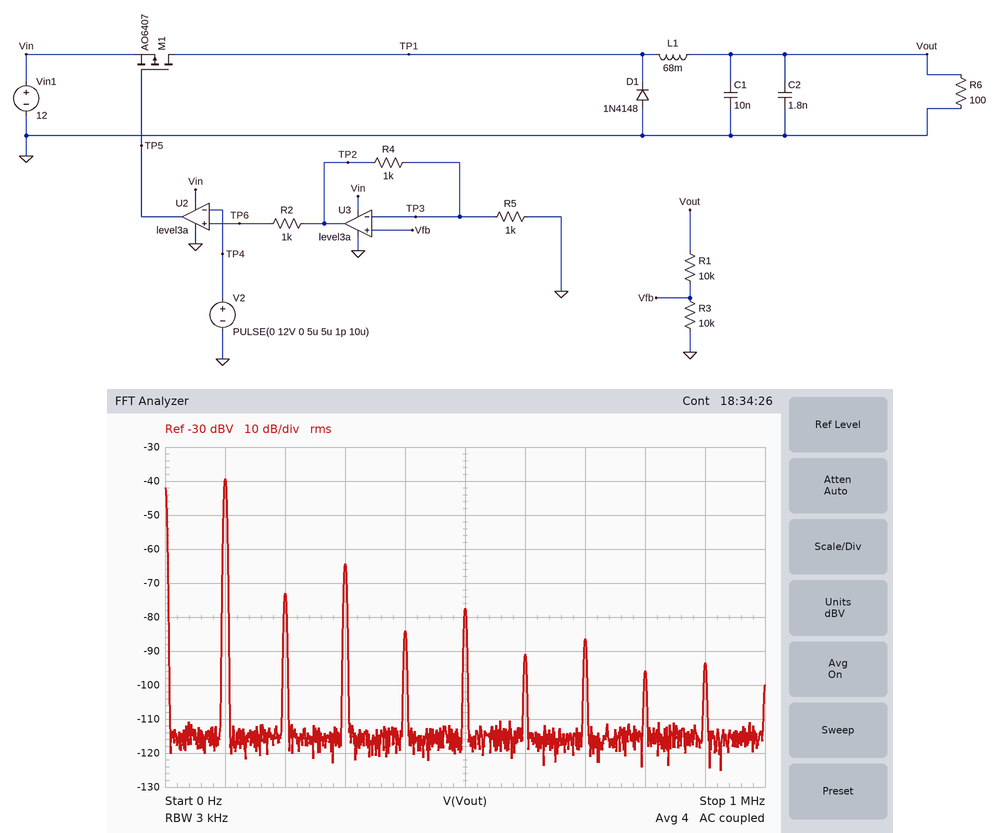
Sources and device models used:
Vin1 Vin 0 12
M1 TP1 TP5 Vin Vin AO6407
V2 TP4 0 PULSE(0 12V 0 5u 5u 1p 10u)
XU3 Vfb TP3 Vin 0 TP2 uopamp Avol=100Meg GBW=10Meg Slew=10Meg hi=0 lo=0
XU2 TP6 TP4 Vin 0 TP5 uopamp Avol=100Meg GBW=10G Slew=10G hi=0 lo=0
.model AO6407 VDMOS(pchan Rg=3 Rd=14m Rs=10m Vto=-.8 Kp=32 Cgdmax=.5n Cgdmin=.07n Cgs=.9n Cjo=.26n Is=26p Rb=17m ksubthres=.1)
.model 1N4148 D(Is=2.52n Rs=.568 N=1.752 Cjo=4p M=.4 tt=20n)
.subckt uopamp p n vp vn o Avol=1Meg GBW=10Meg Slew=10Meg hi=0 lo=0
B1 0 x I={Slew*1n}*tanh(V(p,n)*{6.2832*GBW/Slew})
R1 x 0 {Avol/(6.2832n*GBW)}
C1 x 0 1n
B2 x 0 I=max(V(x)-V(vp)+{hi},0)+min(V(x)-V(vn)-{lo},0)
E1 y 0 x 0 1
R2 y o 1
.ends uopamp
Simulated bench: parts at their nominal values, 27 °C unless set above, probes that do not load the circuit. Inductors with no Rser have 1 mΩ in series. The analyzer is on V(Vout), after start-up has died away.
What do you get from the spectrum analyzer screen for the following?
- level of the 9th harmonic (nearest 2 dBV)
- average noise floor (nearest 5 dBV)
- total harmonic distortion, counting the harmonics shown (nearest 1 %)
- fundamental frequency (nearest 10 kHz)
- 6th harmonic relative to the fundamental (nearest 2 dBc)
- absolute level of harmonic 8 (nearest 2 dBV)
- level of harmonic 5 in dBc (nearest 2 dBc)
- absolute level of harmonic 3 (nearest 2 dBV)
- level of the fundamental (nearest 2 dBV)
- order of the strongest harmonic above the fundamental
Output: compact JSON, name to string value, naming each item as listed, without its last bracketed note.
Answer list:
{"level of the 9th harmonic": "-94 dBV", "average noise floor": "-115 dBV", "total harmonic distortion, counting the harmonics shown": "6 %", "fundamental frequency": "100 kHz", "6th harmonic relative to the fundamental": "-52 dBc", "absolute level of harmonic 8": "-96 dBV", "level of harmonic 5 in dBc": "-38 dBc", "absolute level of harmonic 3": "-64 dBV", "level of the fundamental": "-40 dBV", "order of the strongest harmonic above the fundamental": "3"}
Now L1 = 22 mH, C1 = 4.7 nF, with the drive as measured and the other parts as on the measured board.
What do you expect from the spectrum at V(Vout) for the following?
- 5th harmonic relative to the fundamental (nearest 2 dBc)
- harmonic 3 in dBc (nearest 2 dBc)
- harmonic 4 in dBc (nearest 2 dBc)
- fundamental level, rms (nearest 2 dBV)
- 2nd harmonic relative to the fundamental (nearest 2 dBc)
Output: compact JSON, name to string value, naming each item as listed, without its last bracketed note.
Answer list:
{"5th harmonic relative to the fundamental": "-34 dBc", "harmonic 3 in dBc": "-22 dBc", "harmonic 4 in dBc": "-42 dBc", "fundamental level, rms": "-28 dBV", "2nd harmonic relative to the fundamental": "-32 dBc"}
